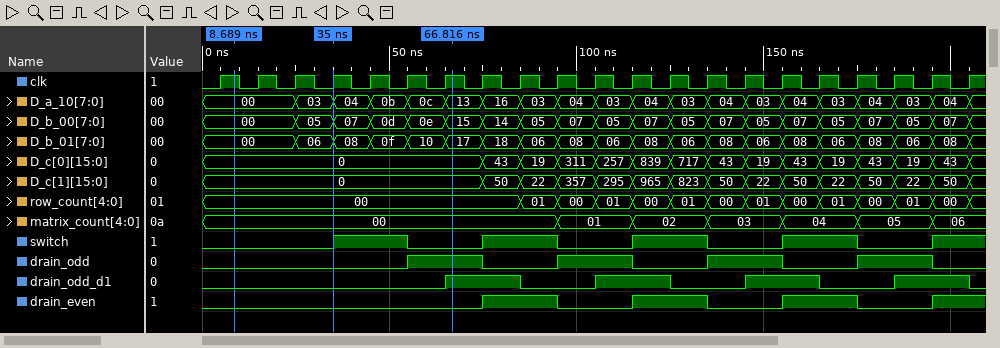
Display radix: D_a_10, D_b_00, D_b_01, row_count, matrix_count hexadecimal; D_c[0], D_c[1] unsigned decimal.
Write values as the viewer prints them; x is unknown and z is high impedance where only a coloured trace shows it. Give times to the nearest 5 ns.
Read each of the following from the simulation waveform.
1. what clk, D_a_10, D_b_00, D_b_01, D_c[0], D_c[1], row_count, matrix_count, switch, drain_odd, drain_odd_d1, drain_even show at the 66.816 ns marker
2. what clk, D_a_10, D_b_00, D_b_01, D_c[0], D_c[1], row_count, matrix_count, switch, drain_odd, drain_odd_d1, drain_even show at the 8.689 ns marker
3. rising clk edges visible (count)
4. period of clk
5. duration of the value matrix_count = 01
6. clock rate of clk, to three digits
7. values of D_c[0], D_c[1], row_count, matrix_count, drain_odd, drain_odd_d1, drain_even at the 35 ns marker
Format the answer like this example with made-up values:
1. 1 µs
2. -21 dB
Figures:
1. clk=1, D_a_10=13, D_b_00=15, D_b_01=17, D_c[0]=0, D_c[1]=0, row_count=00, matrix_count=00, switch=0, drain_odd=1, drain_odd_d1=1, drain_even=0
2. clk=1, D_a_10=00, D_b_00=00, D_b_01=00, D_c[0]=0, D_c[1]=0, row_count=00, matrix_count=00, switch=0, drain_odd=0, drain_odd_d1=0, drain_even=0
3. 21
4. 10 ns
5. 20 ns
6. 100 MHz
7. D_c[0]=0, D_c[1]=0, row_count=00, matrix_count=00, drain_odd=0, drain_odd_d1=0, drain_even=0
